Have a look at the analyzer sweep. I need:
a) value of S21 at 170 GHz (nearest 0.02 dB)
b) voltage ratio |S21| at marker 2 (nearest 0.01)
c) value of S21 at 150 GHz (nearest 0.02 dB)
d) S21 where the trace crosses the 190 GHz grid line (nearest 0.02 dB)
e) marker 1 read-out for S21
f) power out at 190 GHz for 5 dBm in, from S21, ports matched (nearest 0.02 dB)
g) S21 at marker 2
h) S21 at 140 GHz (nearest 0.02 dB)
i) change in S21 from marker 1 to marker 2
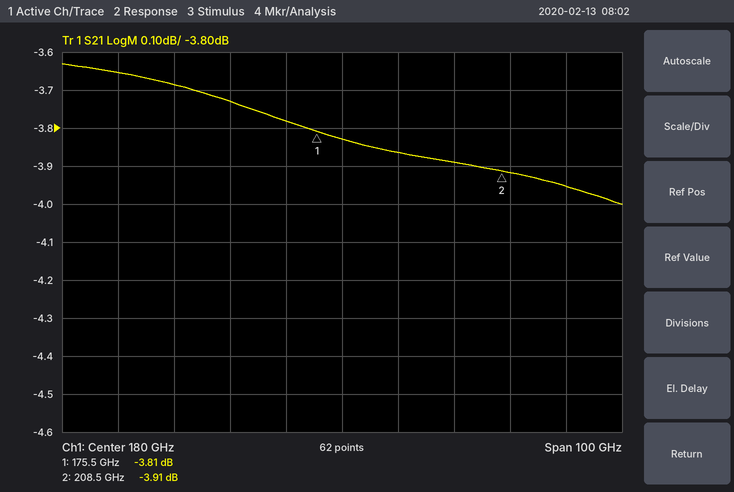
-3.78 dB
0.64
-3.68 dB
-3.86 dB
-3.81 dB
1.14 dBm
-3.91 dB
-3.66 dB
-0.10 dB
